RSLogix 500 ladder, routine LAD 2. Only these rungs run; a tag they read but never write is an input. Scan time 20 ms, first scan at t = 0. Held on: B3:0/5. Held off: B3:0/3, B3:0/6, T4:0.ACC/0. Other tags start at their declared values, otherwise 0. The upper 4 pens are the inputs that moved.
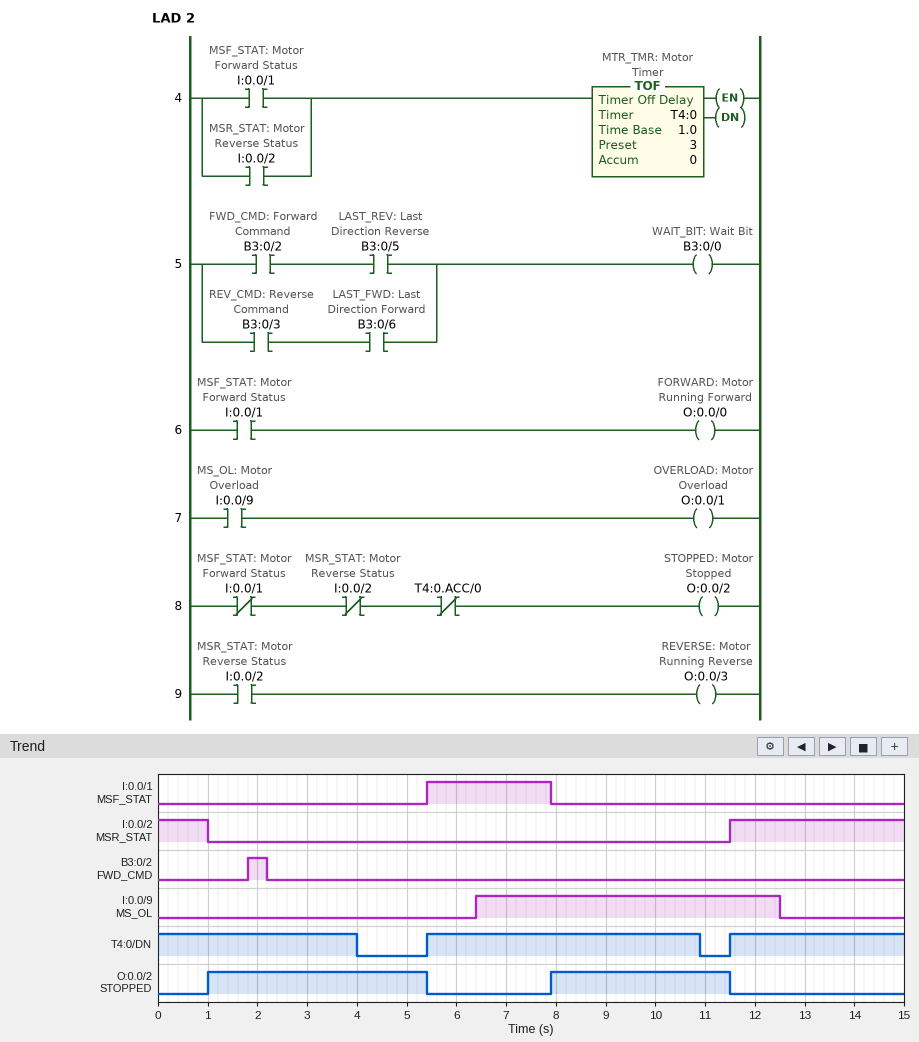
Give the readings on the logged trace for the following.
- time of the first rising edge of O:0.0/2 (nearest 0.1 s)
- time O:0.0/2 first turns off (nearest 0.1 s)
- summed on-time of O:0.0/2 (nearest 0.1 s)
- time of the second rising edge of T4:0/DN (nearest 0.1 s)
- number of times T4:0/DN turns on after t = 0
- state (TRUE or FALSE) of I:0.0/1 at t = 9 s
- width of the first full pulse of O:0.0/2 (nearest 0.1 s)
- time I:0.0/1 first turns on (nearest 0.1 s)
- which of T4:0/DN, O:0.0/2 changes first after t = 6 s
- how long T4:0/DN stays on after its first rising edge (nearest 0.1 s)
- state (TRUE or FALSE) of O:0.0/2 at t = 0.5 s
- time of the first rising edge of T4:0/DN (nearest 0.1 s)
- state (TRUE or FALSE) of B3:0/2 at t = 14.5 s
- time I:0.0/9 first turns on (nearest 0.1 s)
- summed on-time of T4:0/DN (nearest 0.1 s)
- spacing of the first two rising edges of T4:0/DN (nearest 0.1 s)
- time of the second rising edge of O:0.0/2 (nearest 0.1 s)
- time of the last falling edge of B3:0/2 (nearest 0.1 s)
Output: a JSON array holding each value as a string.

["1.0 s", "5.4 s", "8.0 s", "11.5 s", "2", "FALSE", "4.4 s", "5.4 s", "O:0.0/2", "5.5 s", "FALSE", "5.4 s", "FALSE", "6.4 s", "13.0 s", "6.1 s", "7.9 s", "2.2 s"]
